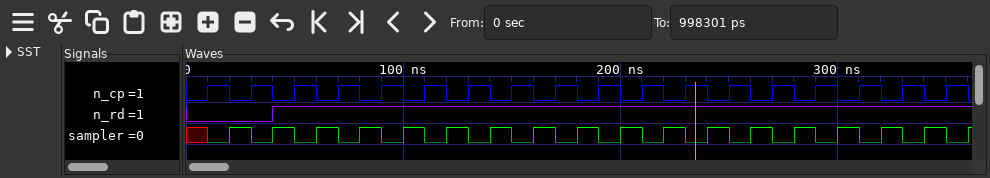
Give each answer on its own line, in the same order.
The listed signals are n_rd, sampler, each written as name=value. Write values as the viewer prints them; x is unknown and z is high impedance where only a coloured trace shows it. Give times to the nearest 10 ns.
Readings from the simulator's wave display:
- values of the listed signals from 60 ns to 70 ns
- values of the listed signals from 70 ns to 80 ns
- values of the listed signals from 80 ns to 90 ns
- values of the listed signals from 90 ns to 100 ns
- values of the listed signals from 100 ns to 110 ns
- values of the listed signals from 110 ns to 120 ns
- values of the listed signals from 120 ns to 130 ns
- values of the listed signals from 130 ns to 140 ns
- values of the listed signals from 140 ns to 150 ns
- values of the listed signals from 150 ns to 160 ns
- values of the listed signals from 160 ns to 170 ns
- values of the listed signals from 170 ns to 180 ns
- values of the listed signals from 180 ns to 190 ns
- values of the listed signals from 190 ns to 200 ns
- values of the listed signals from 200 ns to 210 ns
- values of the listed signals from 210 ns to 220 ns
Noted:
n_rd=1, sampler=1
n_rd=1, sampler=0
n_rd=1, sampler=1
n_rd=1, sampler=0
n_rd=1, sampler=1
n_rd=1, sampler=0
n_rd=1, sampler=1
n_rd=1, sampler=0
n_rd=1, sampler=1
n_rd=1, sampler=0
n_rd=1, sampler=1
n_rd=1, sampler=0
n_rd=1, sampler=1
n_rd=1, sampler=0
n_rd=1, sampler=1
n_rd=1, sampler=0
